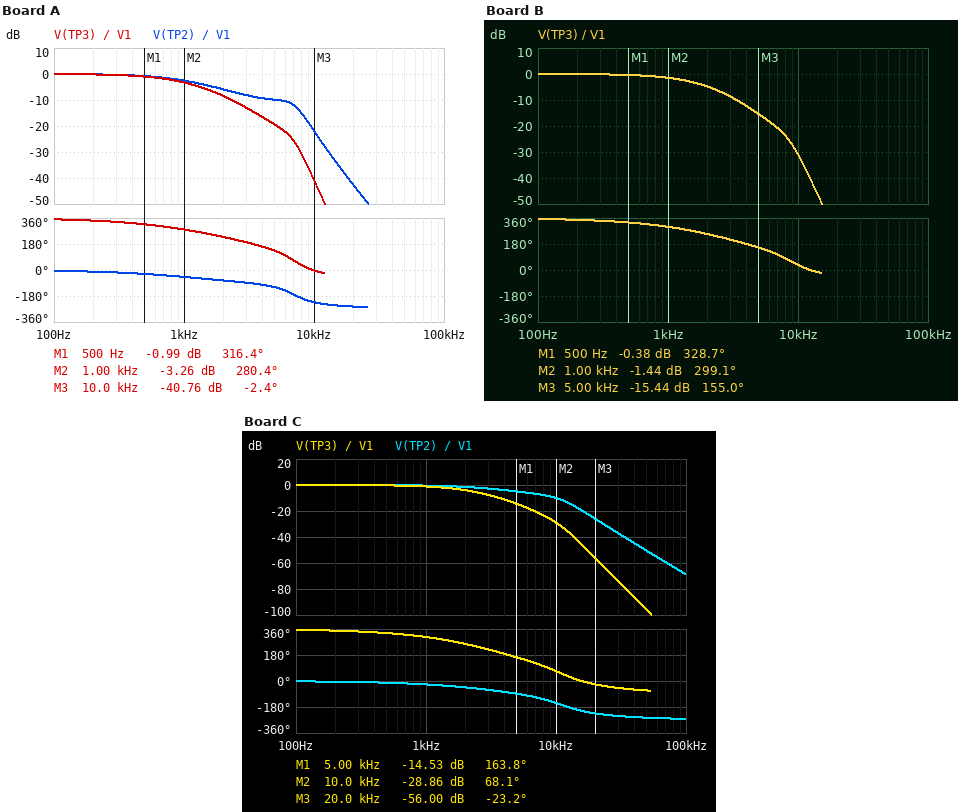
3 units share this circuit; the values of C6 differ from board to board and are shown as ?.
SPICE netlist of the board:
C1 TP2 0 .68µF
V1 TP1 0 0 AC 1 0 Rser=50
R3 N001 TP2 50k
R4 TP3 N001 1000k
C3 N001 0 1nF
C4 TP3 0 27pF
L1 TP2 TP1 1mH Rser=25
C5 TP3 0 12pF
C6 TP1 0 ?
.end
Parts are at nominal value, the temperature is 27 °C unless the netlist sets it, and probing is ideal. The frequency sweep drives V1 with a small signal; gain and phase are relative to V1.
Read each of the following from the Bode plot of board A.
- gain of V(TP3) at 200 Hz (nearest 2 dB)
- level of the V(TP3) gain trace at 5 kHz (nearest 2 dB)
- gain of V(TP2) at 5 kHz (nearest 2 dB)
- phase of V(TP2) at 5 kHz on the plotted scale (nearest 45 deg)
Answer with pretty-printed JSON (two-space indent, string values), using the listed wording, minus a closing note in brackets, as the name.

{
  "gain of V(TP3) at 200 Hz": "0 dB",
  "level of the V(TP3) gain trace at 5 kHz": "-20 dB",
  "gain of V(TP2) at 5 kHz": "-10 dB",
  "phase of V(TP2) at 5 kHz on the plotted scale": "-135 deg"
}
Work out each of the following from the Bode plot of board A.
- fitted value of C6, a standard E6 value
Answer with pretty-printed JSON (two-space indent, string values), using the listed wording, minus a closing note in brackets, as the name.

{
  "fitted value of C6, a standard E6 value": "2.2 µF"
}
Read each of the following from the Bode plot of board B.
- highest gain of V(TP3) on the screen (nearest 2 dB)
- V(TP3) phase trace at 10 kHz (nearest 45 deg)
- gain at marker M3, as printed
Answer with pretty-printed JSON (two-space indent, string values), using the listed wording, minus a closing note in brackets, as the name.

{
  "highest gain of V(TP3) on the screen": "0 dB",
  "V(TP3) phase trace at 10 kHz": "45 deg",
  "gain at marker M3, as printed": "-15.44 dB"
}
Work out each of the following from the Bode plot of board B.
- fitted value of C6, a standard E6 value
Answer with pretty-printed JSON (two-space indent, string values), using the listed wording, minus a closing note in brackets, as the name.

{
  "fitted value of C6, a standard E6 value": "680 nF"
}
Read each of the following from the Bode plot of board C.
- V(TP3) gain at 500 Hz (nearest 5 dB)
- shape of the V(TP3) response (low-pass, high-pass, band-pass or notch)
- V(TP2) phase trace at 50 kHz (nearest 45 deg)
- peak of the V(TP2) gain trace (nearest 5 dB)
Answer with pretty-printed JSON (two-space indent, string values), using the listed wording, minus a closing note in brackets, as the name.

{
  "V(TP3) gain at 500 Hz": "0 dB",
  "shape of the V(TP3) response": "low-pass",
  "V(TP2) phase trace at 50 kHz": "-270 deg",
  "peak of the V(TP2) gain trace": "0 dB"
}
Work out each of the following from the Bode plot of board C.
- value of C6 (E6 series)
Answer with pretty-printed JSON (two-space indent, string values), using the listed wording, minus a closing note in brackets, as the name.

{
  "value of C6": "330 nF"
}
